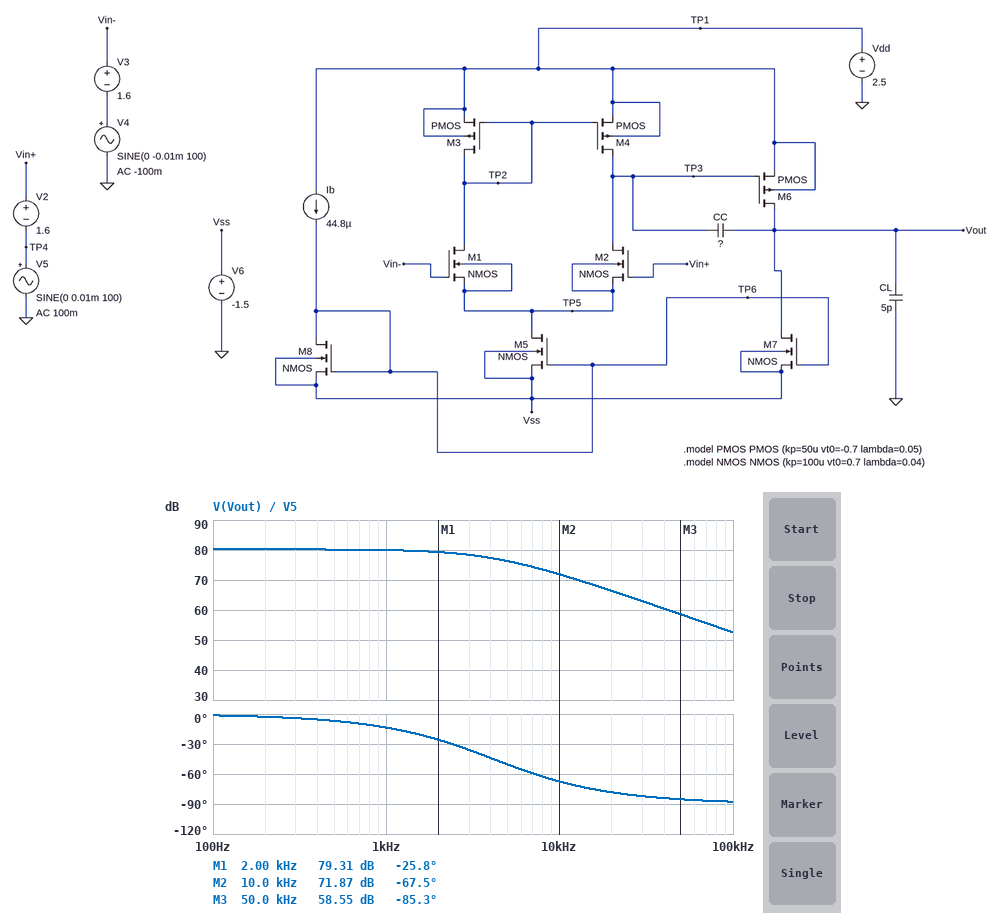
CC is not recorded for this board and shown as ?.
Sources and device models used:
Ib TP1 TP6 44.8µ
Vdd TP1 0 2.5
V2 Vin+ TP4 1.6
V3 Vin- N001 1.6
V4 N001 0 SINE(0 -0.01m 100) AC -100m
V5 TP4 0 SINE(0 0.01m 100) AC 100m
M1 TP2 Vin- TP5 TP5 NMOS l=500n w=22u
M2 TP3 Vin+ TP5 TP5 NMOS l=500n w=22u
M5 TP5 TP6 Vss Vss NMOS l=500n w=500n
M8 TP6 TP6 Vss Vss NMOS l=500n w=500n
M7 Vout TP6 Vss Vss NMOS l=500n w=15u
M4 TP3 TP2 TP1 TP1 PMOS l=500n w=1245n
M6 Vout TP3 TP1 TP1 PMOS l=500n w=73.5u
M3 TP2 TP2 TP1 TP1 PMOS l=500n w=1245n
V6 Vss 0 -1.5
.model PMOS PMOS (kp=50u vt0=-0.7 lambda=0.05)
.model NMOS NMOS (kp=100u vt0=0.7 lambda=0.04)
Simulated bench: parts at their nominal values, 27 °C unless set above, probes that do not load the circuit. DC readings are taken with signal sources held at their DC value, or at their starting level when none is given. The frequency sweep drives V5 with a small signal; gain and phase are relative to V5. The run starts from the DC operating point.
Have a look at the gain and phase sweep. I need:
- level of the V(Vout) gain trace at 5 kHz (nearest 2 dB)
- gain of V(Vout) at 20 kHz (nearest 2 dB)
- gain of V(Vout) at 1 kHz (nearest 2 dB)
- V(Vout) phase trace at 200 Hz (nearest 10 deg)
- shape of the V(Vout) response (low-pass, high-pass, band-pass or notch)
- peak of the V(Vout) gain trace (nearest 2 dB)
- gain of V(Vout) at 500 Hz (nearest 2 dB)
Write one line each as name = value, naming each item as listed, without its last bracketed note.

level of the V(Vout) gain trace at 5 kHz = 76 dB
gain of V(Vout) at 20 kHz = 66 dB
gain of V(Vout) at 1 kHz = 80 dB
V(Vout) phase trace at 200 Hz = 0 deg
shape of the V(Vout) response = low-pass
peak of the V(Vout) gain trace = 80 dB
gain of V(Vout) at 500 Hz = 80 dB
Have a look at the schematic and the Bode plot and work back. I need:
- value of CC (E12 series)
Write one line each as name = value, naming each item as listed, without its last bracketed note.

value of CC = 1.8 pF
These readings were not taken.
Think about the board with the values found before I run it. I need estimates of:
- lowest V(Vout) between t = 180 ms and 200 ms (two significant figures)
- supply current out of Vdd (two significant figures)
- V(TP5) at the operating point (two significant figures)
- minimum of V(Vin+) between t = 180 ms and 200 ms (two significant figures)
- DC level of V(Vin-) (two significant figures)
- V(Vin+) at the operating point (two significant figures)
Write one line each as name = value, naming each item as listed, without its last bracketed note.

lowest V(Vout) between t = 180 ms and 200 ms = 650 mV
supply current out of Vdd = 1.5 mA
V(TP5) at the operating point = 800 mV
minimum of V(Vin+) between t = 180 ms and 200 ms = 1.6 V
DC level of V(Vin-) = 1.6 V
V(Vin+) at the operating point = 1.6 V
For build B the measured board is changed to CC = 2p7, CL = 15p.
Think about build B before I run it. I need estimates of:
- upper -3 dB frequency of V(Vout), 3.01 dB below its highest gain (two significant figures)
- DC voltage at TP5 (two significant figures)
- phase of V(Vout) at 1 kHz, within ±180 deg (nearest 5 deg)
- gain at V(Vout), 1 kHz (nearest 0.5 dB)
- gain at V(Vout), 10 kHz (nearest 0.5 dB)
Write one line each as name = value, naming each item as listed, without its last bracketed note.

upper -3 dB frequency of V(Vout), 3.01 dB below its highest gain = 2.8 kHz
DC voltage at TP5 = 800 mV
phase of V(Vout) at 1 kHz, within ±180 deg = -20 deg
gain at V(Vout), 1 kHz = 79.5 dB
gain at V(Vout), 10 kHz = 68.5 dB
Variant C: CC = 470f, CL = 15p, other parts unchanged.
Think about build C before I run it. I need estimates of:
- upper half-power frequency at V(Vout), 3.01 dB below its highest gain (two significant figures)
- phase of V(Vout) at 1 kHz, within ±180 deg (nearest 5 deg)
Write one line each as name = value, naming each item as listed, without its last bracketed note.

upper half-power frequency at V(Vout), 3.01 dB below its highest gain = 16 kHz
phase of V(Vout) at 1 kHz, within ±180 deg = -5 deg
